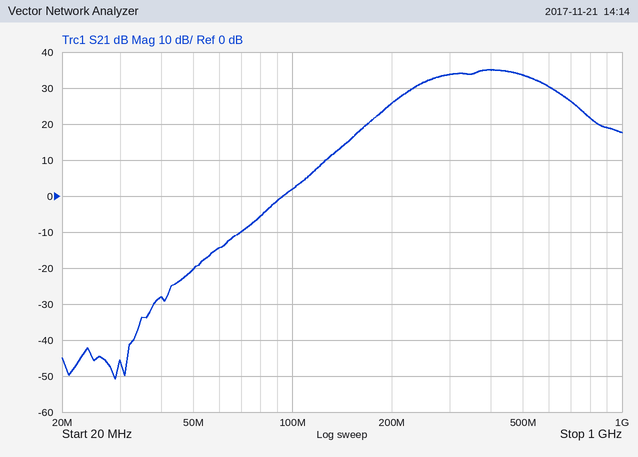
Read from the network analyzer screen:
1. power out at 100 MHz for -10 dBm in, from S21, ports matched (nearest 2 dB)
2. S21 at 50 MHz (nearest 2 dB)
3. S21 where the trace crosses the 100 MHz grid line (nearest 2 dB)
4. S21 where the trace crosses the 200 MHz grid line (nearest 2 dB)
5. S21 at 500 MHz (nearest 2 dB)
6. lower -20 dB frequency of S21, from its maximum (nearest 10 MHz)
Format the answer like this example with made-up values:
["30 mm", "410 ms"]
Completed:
["-8 dBm", "-20 dB", "2 dB", "26 dB", "34 dB", "150 MHz"]
